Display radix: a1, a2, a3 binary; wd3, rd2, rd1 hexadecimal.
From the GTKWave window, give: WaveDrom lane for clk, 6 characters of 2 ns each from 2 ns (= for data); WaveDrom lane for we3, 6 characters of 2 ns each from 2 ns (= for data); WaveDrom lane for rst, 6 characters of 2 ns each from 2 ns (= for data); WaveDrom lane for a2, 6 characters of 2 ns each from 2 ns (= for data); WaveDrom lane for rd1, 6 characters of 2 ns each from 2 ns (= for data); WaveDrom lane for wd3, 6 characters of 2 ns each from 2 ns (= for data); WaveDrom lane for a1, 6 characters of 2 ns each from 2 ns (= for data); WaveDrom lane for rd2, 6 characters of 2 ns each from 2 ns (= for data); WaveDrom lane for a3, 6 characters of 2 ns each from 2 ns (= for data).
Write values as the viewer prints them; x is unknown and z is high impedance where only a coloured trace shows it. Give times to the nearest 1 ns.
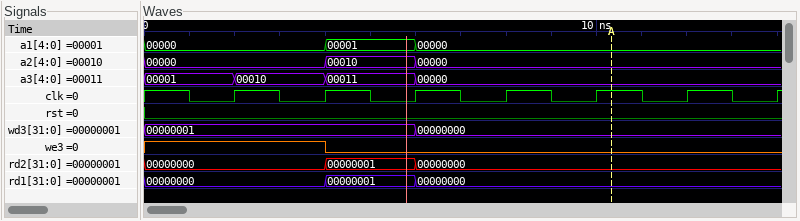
{name: 'clk', wave: 'p.....'}
{name: 'we3', wave: '10....'}
{name: 'rst', wave: '0.....'}
{name: 'a2', wave: '===...', data: '00000 00010 00000'}
{name: 'rd1', wave: '===...', data: '00000000 00000001 00000000'}
{name: 'wd3', wave: '=.=...', data: '00000001 00000000'}
{name: 'a1', wave: '===...', data: '00000 00001 00000'}
{name: 'rd2', wave: '===...', data: '00000000 00000001 00000000'}
{name: 'a3', wave: '===...', data: '00010 00011 00000'}
